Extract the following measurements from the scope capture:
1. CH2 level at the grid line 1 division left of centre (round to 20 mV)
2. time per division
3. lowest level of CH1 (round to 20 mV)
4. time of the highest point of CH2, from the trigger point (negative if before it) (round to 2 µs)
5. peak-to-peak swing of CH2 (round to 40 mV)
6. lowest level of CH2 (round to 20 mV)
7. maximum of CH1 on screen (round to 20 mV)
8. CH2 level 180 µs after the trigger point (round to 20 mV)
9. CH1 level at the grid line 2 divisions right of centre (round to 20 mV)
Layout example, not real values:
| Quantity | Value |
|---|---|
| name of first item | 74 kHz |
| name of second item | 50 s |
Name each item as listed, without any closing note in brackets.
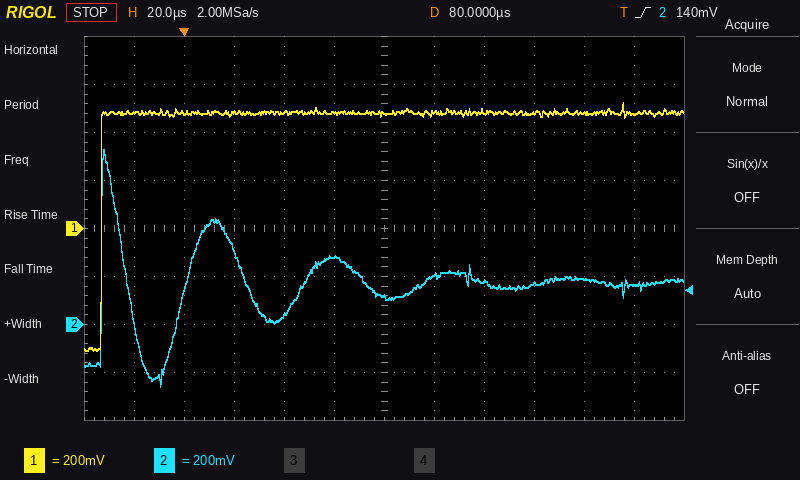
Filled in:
| Quantity | Value |
|---|---|
| CH2 level at the grid line 1 division left of centre | 280 mV |
| time per division | 20 µs |
| lowest level of CH1 | -500 mV |
| time of the highest point of CH2, from the trigger point (negative if before it) | -32 µs |
| peak-to-peak swing of CH2 | 1.00 V |
| lowest level of CH2 | -260 mV |
| maximum of CH1 on screen | 520 mV |
| CH2 level 180 µs after the trigger point | 160 mV |
| CH1 level at the grid line 2 divisions right of centre | 480 mV |
